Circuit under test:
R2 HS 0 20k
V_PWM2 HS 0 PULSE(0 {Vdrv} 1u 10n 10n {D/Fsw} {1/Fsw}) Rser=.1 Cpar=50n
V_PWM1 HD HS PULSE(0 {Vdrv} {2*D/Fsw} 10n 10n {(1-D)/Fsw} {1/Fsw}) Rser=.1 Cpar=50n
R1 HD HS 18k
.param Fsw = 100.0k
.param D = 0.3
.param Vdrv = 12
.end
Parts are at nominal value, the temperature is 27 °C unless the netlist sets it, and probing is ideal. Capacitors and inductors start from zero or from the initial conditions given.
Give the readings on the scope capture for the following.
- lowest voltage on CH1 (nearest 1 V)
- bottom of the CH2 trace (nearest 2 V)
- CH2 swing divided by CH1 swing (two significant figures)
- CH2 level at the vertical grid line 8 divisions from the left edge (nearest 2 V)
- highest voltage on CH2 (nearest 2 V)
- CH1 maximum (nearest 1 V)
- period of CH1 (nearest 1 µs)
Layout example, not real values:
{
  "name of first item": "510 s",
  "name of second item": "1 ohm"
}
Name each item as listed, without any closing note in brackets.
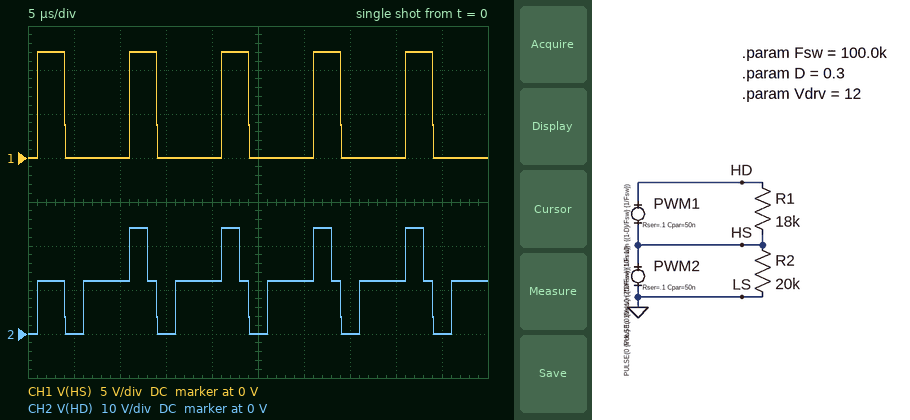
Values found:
{
  "lowest voltage on CH1": "0 V",
  "bottom of the CH2 trace": "0 V",
  "CH2 swing divided by CH1 swing": "2.0",
  "CH2 level at the vertical grid line 8 divisions from the left edge": "12 V",
  "highest voltage on CH2": "24 V",
  "CH1 maximum": "12 V",
  "period of CH1": "10 µs"
}
